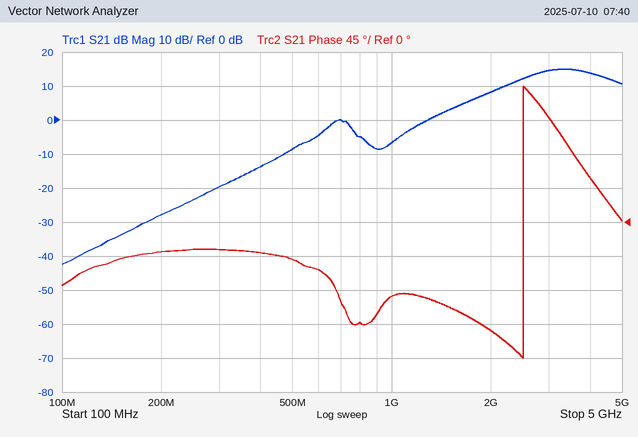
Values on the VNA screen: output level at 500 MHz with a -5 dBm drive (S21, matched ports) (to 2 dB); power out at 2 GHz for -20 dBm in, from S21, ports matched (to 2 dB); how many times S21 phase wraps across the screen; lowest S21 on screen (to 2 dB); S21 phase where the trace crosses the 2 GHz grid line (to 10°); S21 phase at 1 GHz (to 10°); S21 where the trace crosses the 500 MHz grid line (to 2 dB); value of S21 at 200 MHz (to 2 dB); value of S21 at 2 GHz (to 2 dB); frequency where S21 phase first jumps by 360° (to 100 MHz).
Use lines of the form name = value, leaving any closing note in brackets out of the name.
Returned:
output level at 500 MHz with a -5 dBm drive (S21, matched ports) = -14 dBm
power out at 2 GHz for -20 dBm in, from S21, ports matched = -12 dBm
how many times S21 phase wraps across the screen = 1
lowest S21 on screen = -42 dB
S21 phase where the trace crosses the 2 GHz grid line = -140°
S21 phase at 1 GHz = -100°
S21 where the trace crosses the 500 MHz grid line = -8 dB
value of S21 at 200 MHz = -28 dB
value of S21 at 2 GHz = 8 dB
frequency where S21 phase first jumps by 360° = 2.5 GHz
